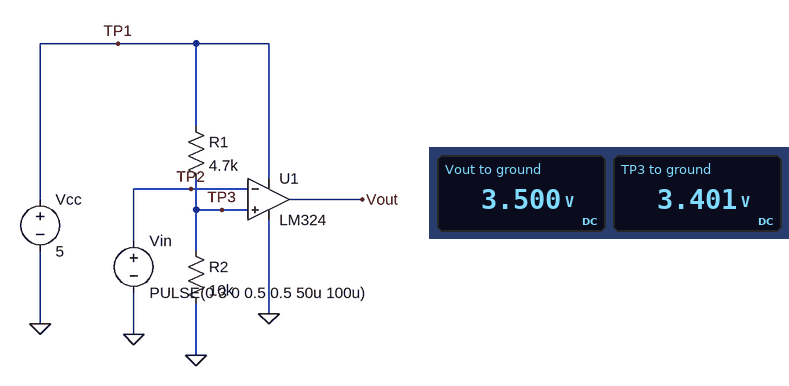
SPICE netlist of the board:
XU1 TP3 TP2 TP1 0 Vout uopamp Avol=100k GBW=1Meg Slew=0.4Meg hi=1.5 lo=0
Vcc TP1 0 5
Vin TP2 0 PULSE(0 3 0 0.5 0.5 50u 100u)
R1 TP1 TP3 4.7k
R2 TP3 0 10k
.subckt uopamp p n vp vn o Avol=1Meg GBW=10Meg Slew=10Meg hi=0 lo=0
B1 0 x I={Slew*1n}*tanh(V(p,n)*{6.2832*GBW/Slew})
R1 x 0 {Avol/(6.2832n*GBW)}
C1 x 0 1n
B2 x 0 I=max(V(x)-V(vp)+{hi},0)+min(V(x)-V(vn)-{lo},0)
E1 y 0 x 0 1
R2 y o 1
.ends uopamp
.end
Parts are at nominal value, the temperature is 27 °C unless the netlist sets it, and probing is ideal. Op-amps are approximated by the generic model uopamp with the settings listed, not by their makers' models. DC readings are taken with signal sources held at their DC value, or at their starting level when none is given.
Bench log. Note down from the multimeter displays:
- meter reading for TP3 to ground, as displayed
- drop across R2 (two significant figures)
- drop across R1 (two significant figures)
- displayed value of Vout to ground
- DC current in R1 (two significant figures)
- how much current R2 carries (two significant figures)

3.401 V
3.4 V
1.6 V
3.500 V
340 µA
340 µA
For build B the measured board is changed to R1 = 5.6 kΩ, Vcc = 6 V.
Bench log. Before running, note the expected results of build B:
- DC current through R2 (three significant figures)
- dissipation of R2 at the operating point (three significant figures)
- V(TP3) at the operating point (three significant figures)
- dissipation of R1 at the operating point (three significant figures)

385 µA
1.48 mW
3.85 V
828 µW
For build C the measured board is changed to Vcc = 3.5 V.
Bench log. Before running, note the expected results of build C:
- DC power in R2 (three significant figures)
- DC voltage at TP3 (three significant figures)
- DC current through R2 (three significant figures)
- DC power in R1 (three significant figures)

567 µW
2.38 V
238 µA
266 µW
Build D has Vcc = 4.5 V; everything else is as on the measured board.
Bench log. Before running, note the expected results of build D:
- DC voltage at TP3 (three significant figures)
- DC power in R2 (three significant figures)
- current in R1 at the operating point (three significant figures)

3.06 V
937 µW
306 µA
